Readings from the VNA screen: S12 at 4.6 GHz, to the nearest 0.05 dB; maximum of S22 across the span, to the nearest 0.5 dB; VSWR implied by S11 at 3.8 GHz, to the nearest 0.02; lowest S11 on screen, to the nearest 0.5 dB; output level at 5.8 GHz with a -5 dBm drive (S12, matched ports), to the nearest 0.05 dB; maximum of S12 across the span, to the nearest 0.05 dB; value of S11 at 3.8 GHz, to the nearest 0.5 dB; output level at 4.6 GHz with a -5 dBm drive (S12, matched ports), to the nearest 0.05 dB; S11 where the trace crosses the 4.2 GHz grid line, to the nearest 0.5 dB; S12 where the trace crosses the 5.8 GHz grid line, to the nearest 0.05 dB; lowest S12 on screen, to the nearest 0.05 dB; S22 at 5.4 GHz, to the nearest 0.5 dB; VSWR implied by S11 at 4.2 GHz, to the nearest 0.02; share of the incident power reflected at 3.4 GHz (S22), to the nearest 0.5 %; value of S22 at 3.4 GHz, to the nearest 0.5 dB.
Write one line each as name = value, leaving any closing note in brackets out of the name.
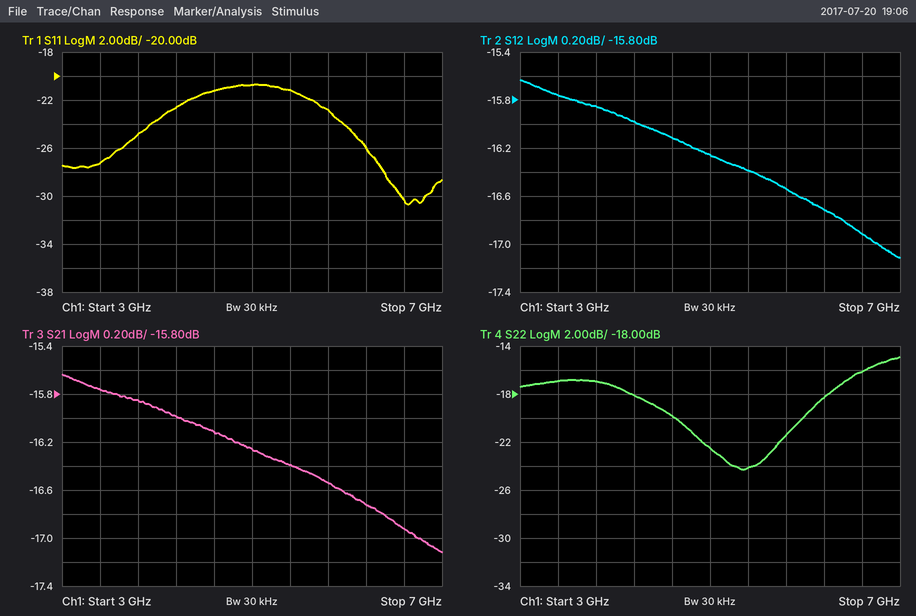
S12 at 4.6 GHz, to the nearest 0.05 dB = -16.10 dB
maximum of S22 across the span, to the nearest 0.5 dB = -15.0 dB
VSWR implied by S11 at 3.8 GHz, to the nearest 0.02 = 1.12
lowest S11 on screen, to the nearest 0.5 dB = -30.5 dB
output level at 5.8 GHz with a -5 dBm drive (S12, matched ports), to the nearest 0.05 dB = -21.55 dBm
maximum of S12 across the span, to the nearest 0.05 dB = -15.65 dB
value of S11 at 3.8 GHz, to the nearest 0.5 dB = -25.0 dB
output level at 4.6 GHz with a -5 dBm drive (S12, matched ports), to the nearest 0.05 dB = -21.10 dBm
S11 where the trace crosses the 4.2 GHz grid line, to the nearest 0.5 dB = -22.5 dB
S12 where the trace crosses the 5.8 GHz grid line, to the nearest 0.05 dB = -16.55 dB
lowest S12 on screen, to the nearest 0.05 dB = -17.10 dB
S22 at 5.4 GHz, to the nearest 0.5 dB = -24.0 dB
VSWR implied by S11 at 4.2 GHz, to the nearest 0.02 = 1.16
share of the incident power reflected at 3.4 GHz (S22), to the nearest 0.5 % = 2.0 %
value of S22 at 3.4 GHz, to the nearest 0.5 dB = -17.0 dB
